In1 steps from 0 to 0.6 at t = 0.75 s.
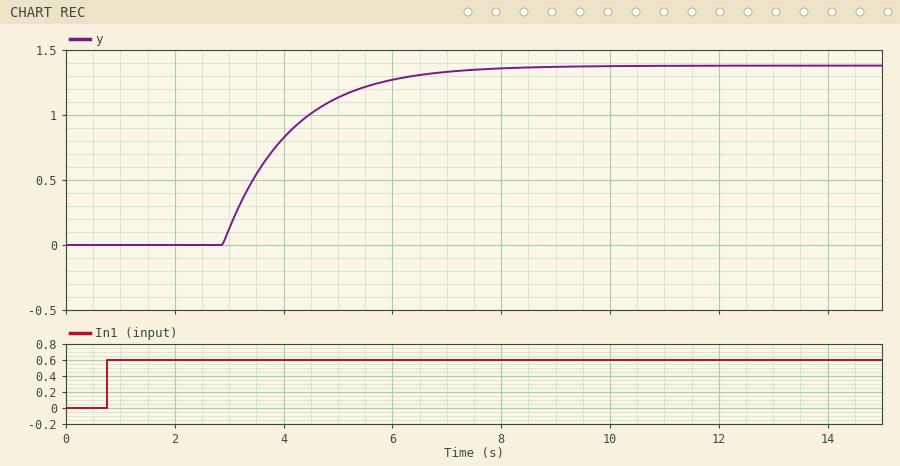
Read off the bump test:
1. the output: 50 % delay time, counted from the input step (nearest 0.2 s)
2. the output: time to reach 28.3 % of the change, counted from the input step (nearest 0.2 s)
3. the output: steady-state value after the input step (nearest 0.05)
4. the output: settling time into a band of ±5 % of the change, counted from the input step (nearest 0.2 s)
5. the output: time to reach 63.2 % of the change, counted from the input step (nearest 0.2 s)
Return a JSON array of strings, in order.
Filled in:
["3.0 s", "2.6 s", "1.40", "5.8 s", "3.4 s"]
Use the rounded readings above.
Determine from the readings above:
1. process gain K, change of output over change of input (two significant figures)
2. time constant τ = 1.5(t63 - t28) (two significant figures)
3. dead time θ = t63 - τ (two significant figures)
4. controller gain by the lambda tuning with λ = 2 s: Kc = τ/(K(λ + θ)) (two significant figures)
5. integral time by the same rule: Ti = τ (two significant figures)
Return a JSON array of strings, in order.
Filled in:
["2.3", "1.2 s", "2.2 s", "0.12", "1.2 s"]
